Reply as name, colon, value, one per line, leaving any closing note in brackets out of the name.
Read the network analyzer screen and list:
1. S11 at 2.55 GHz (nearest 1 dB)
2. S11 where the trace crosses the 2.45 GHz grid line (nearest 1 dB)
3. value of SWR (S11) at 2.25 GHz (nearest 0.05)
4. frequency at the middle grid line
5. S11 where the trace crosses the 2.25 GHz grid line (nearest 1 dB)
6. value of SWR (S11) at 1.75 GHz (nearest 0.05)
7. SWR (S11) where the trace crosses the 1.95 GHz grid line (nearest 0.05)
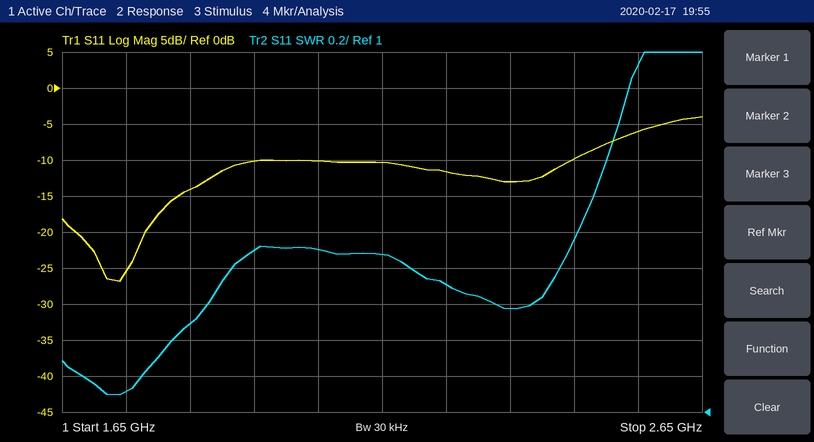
S11 at 2.55 GHz: -6 dB
S11 where the trace crosses the 2.45 GHz grid line: -10 dB
value of SWR (S11) at 2.25 GHz: 1.70
frequency at the middle grid line: 2.15 GHz
S11 where the trace crosses the 2.25 GHz grid line: -12 dB
value of SWR (S11) at 1.75 GHz: 1.10
SWR (S11) where the trace crosses the 1.95 GHz grid line: 1.90
